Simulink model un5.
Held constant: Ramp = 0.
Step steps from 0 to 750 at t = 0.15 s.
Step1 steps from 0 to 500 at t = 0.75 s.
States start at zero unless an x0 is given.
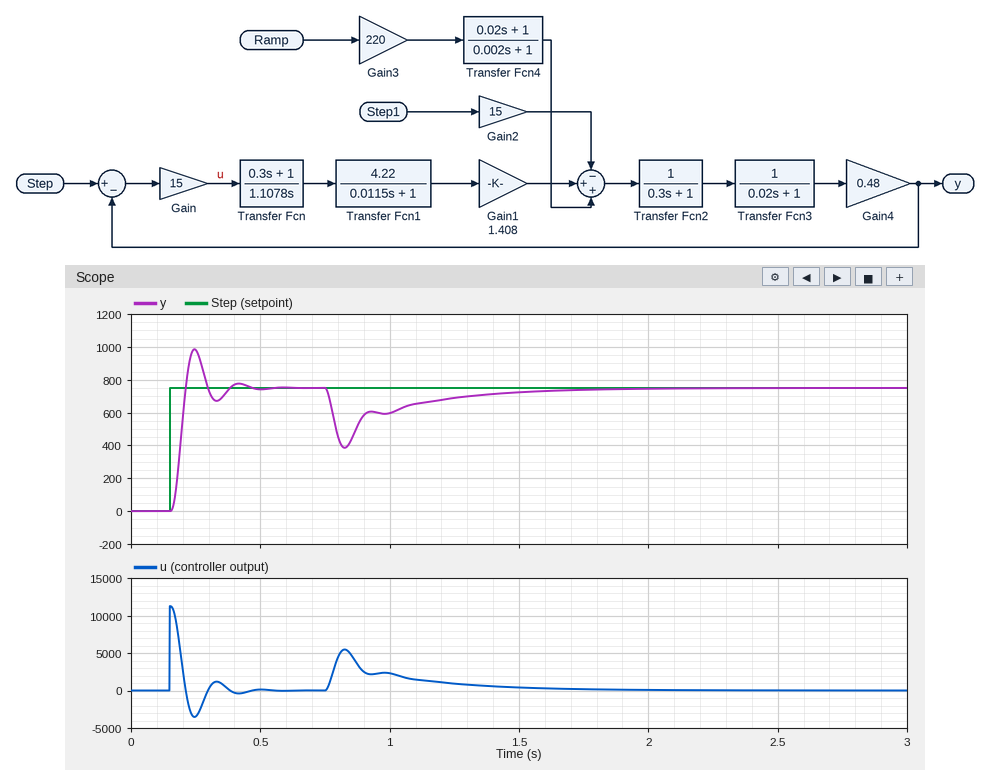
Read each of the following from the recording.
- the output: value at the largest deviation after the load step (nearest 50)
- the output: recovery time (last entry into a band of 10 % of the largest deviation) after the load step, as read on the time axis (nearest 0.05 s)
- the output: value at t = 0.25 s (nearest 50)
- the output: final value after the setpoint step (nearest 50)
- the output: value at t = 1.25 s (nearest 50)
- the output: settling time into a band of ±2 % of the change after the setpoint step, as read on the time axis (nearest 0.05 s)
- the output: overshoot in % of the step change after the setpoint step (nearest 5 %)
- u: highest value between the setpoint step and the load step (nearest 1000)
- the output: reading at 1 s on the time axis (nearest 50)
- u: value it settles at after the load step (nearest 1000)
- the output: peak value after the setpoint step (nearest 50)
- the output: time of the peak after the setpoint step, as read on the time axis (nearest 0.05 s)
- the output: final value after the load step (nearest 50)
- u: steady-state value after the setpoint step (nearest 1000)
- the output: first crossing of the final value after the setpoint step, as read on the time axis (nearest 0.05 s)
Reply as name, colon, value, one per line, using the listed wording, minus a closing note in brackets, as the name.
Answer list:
the output: value at the largest deviation after the load step: 400
the output: recovery time (last entry into a band of 10 % of the largest deviation) after the load step, as read on the time axis: 1.40 s
the output: value at t = 0.25 s: 1000
the output: final value after the setpoint step: 750
the output: value at t = 1.25 s: 700
the output: settling time into a band of ±2 % of the change after the setpoint step, as read on the time axis: 0.45 s
the output: overshoot in % of the step change after the setpoint step: 30 %
u: highest value between the setpoint step and the load step: 11000
the output: reading at 1 s on the time axis: 600
u: value it settles at after the load step: 0
the output: peak value after the setpoint step: 1000
the output: time of the peak after the setpoint step, as read on the time axis: 0.25 s
the output: final value after the load step: 750
u: steady-state value after the setpoint step: 0
the output: first crossing of the final value after the setpoint step, as read on the time axis: 0.20 s
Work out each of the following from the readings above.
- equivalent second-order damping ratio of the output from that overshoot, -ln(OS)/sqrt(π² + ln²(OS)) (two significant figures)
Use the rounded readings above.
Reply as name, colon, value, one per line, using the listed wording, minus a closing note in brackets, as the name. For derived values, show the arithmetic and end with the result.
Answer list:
equivalent second-order damping ratio of the output from that overshoot, -ln(OS)/sqrt(π² + ln²(OS)): ln(0.3) = -1.204; 1.204 / sqrt(9.870 + 1.450) = 0.36
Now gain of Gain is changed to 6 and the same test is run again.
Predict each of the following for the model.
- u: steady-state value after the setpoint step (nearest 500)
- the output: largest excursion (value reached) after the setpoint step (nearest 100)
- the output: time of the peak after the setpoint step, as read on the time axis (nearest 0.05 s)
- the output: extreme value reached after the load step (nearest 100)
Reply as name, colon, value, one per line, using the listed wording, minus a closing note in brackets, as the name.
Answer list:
u: steady-state value after the setpoint step: 0
the output: largest excursion (value reached) after the setpoint step: 800
the output: time of the peak after the setpoint step, as read on the time axis: 0.35 s
the output: extreme value reached after the load step: 100
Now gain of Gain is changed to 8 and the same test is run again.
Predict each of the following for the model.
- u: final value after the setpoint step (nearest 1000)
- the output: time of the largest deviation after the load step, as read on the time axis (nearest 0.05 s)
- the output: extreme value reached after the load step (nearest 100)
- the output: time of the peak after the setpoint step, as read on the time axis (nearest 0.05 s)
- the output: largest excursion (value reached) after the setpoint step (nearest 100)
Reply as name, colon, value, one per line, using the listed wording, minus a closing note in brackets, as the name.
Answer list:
u: final value after the setpoint step: 0
the output: time of the largest deviation after the load step, as read on the time axis: 0.85 s
the output: extreme value reached after the load step: 200
the output: time of the peak after the setpoint step, as read on the time axis: 0.30 s
the output: largest excursion (value reached) after the setpoint step: 800
